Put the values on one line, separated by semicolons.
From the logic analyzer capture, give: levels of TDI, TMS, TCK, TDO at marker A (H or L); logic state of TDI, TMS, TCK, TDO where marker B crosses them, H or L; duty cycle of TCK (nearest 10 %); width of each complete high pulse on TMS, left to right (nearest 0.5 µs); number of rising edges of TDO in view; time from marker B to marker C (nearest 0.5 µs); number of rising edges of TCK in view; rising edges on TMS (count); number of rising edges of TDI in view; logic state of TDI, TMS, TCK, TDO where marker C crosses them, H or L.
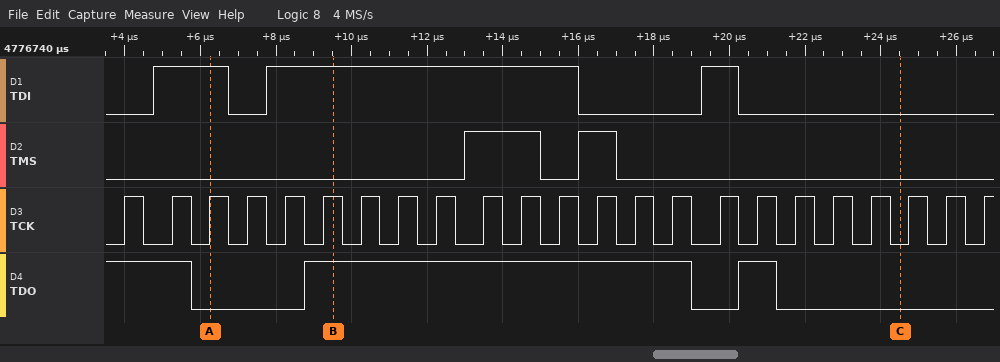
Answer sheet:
TDI=H, TMS=L, TCK=H, TDO=L; TDI=H, TMS=L, TCK=H, TDO=H; 50 %; 2 µs, 1 µs; 2; 15 µs; 23; 2; 3; TDI=L, TMS=L, TCK=L, TDO=L
